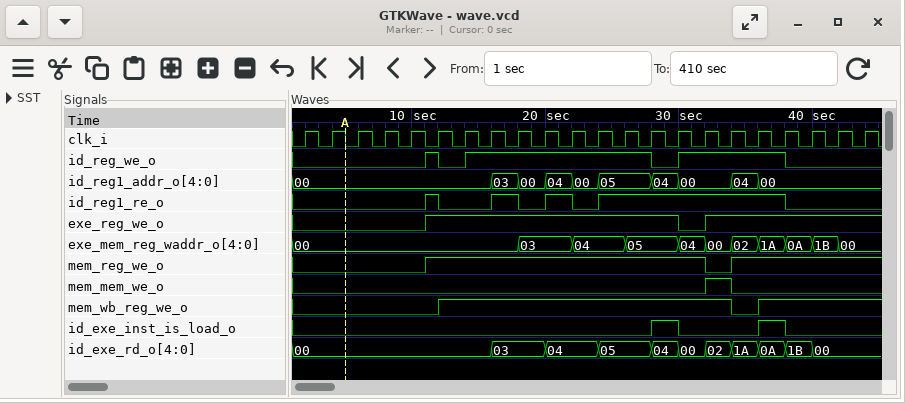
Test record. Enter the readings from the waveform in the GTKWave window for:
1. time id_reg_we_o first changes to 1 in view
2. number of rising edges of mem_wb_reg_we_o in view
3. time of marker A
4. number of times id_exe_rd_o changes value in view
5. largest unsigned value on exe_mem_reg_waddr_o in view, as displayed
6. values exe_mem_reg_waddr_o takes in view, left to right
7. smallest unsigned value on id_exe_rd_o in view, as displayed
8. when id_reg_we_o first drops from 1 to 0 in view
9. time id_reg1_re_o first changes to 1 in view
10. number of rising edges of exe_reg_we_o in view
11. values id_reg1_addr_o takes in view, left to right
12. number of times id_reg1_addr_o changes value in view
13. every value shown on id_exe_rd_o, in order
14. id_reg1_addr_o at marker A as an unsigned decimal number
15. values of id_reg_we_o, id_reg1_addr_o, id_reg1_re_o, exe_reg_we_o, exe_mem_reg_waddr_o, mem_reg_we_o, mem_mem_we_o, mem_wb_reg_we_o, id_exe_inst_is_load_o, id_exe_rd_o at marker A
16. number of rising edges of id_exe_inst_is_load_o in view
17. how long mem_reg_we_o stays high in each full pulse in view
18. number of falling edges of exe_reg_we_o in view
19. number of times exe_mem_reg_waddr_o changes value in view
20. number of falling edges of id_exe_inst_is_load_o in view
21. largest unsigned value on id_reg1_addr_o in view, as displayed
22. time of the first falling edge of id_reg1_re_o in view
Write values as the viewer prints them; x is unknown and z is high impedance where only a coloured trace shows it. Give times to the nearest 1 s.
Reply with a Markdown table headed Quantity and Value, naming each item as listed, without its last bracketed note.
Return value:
| Quantity | Value |
|---|---|
| time id_reg_we_o first changes to 1 in view | 11 s |
| number of rising edges of mem_wb_reg_we_o in view | 2 |
| time of marker A | 5 s |
| number of times id_exe_rd_o changes value in view | 10 |
| largest unsigned value on exe_mem_reg_waddr_o in view, as displayed | 1B |
| values exe_mem_reg_waddr_o takes in view, left to right | 00, 03, 04, 05, 04, 00, 02, 1A, 0A, 1B, 00 |
| smallest unsigned value on id_exe_rd_o in view, as displayed | 00 |
| when id_reg_we_o first drops from 1 to 0 in view | 12 s |
| time id_reg1_re_o first changes to 1 in view | 11 s |
| number of rising edges of exe_reg_we_o in view | 2 |
| values id_reg1_addr_o takes in view, left to right | 00, 03, 00, 04, 00, 05, 04, 00, 04, 00 |
| number of times id_reg1_addr_o changes value in view | 9 |
| every value shown on id_exe_rd_o, in order | 00, 03, 04, 05, 04, 00, 02, 1A, 0A, 1B, 00 |
| id_reg1_addr_o at marker A as an unsigned decimal number | 0 |
| values of id_reg_we_o, id_reg1_addr_o, id_reg1_re_o, exe_reg_we_o, exe_mem_reg_waddr_o, mem_reg_we_o, mem_mem_we_o, mem_wb_reg_we_o, id_exe_inst_is_load_o, id_exe_rd_o at marker A | id_reg_we_o=0, id_reg1_addr_o=00, id_reg1_re_o=0, exe_reg_we_o=0, exe_mem_reg_waddr_o=00, mem_reg_we_o=0, mem_mem_we_o=0, mem_wb_reg_we_o=0, id_exe_inst_is_load_o=0, id_exe_rd_o=00 |
| number of rising edges of id_exe_inst_is_load_o in view | 2 |
| how long mem_reg_we_o stays high in each full pulse in view | 21 s |
| number of falling edges of exe_reg_we_o in view | 1 |
| number of times exe_mem_reg_waddr_o changes value in view | 10 |
| number of falling edges of id_exe_inst_is_load_o in view | 2 |
| largest unsigned value on id_reg1_addr_o in view, as displayed | 05 |
| time of the first falling edge of id_reg1_re_o in view | 12 s |
